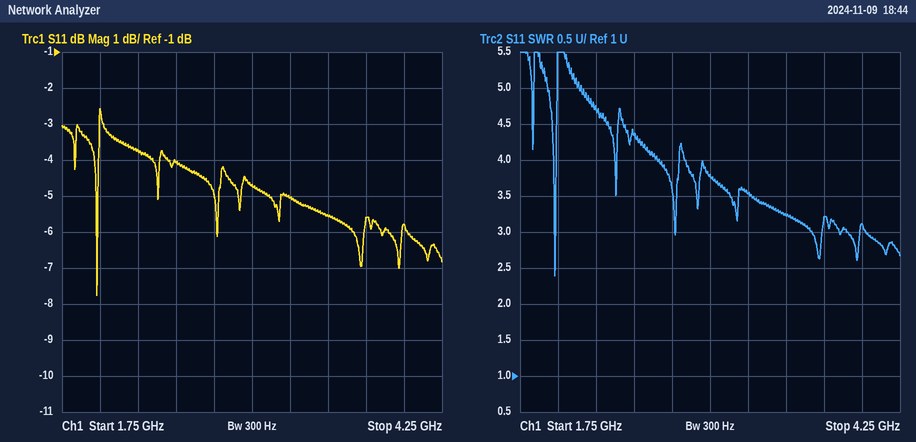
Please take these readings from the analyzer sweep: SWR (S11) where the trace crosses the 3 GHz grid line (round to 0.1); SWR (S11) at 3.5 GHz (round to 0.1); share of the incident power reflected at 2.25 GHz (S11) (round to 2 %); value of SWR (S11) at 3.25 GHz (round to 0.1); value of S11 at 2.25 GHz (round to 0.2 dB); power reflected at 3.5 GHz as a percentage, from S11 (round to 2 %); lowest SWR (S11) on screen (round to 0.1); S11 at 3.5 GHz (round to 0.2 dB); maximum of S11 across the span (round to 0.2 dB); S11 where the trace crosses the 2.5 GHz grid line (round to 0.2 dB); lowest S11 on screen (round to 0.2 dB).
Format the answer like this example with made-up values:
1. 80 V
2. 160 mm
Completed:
1. 3.8
2. 3.2
3. 42 %
4. 3.5
5. -3.8 dB
6. 28 %
7. 2.4
8. -5.6 dB
9. -2.6 dB
10. -4.0 dB
11. -7.8 dB
